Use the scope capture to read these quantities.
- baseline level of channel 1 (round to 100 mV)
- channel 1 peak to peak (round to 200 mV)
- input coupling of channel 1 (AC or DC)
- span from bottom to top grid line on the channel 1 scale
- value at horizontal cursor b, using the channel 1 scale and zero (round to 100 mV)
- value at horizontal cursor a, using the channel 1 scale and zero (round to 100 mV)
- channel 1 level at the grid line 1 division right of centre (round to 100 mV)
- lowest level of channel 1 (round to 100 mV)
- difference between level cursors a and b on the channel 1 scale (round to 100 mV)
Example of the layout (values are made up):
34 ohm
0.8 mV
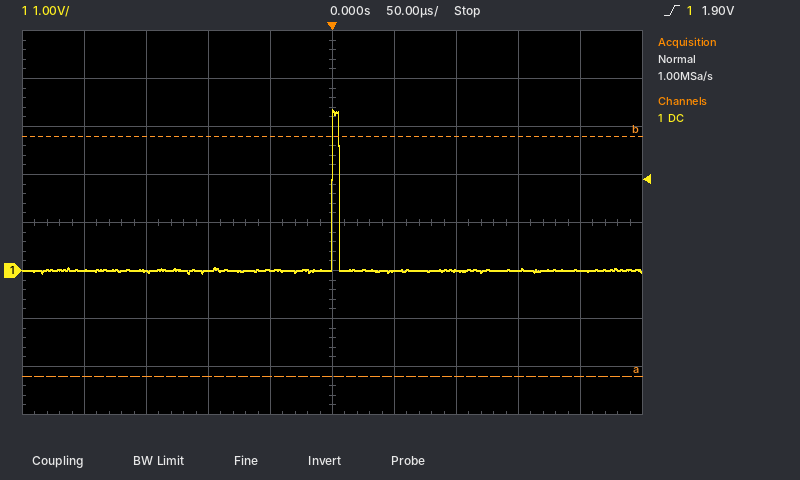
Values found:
0.0 V
3.4 V
DC
8 V
2.8 V
-2.2 V
0.0 V
-100 mV
5.0 V
